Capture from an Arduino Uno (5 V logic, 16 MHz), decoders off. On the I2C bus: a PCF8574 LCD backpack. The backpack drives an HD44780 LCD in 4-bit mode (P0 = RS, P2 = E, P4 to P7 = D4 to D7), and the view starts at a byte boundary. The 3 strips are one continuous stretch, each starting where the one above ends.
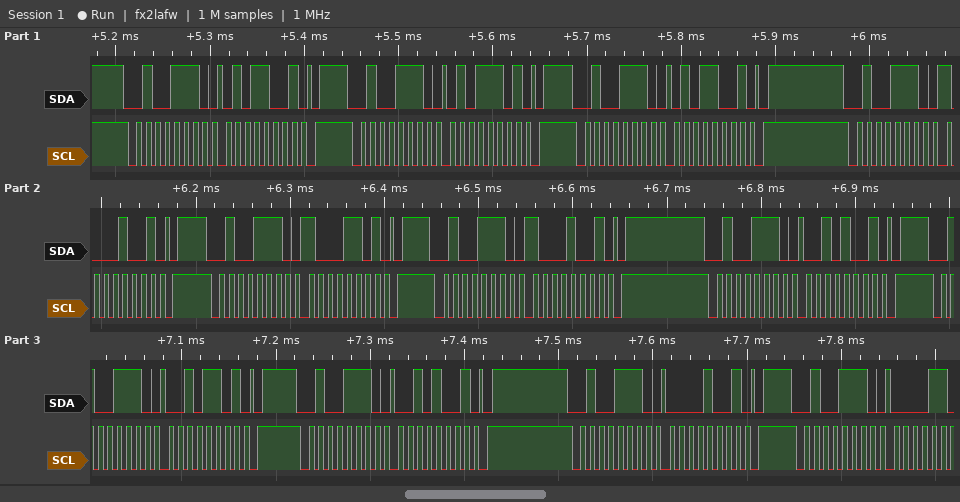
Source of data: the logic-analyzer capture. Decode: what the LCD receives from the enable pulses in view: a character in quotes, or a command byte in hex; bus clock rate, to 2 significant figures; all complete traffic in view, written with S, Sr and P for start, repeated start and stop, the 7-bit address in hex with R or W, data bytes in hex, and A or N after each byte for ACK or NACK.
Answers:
'X'
100 kHz
S 27W A 59 A P S 27W A 5D A P S 27W A 59 A P S 27W A 89 A P S 27W A 8D A P S 27W A 89 A P S 27W A 29 A P S 27W A 2D A P S 27W A 29 A P S 27W A 09 A P S 27W A
